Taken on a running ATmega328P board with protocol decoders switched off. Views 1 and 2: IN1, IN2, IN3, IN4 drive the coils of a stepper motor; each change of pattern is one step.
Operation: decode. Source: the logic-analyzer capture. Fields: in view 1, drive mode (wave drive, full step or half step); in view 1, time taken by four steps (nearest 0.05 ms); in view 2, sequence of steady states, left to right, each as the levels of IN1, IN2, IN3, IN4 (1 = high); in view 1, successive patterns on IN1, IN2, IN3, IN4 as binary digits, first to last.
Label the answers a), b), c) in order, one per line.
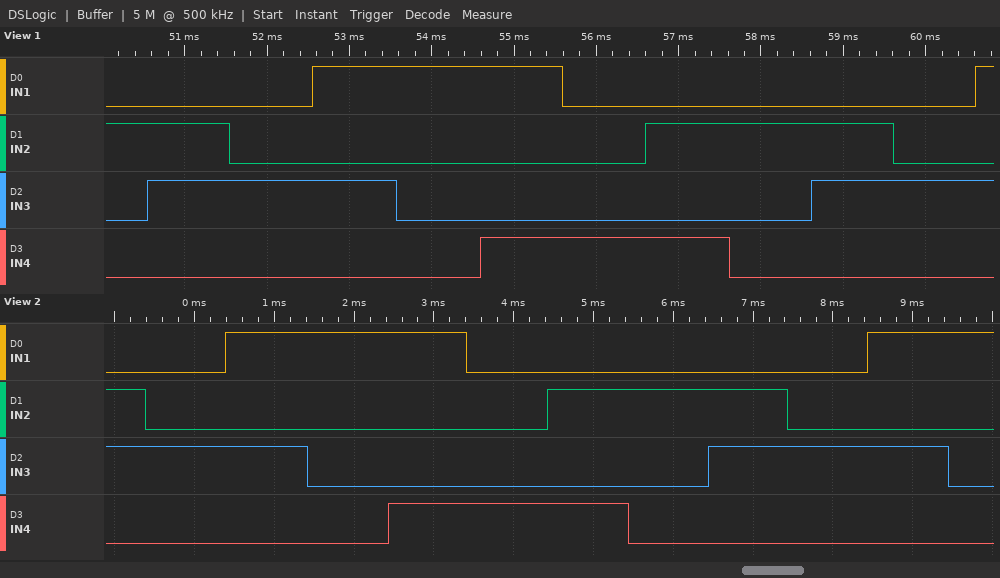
a) half step
b) 4.05 ms
c) 0110 0010 1010 1000 1001 0001 0101 0100 0110 0010 1010 1000
d) 0100 0110 0010 1010 1000 1001 0001 0101 0100 0110 0010 1010
